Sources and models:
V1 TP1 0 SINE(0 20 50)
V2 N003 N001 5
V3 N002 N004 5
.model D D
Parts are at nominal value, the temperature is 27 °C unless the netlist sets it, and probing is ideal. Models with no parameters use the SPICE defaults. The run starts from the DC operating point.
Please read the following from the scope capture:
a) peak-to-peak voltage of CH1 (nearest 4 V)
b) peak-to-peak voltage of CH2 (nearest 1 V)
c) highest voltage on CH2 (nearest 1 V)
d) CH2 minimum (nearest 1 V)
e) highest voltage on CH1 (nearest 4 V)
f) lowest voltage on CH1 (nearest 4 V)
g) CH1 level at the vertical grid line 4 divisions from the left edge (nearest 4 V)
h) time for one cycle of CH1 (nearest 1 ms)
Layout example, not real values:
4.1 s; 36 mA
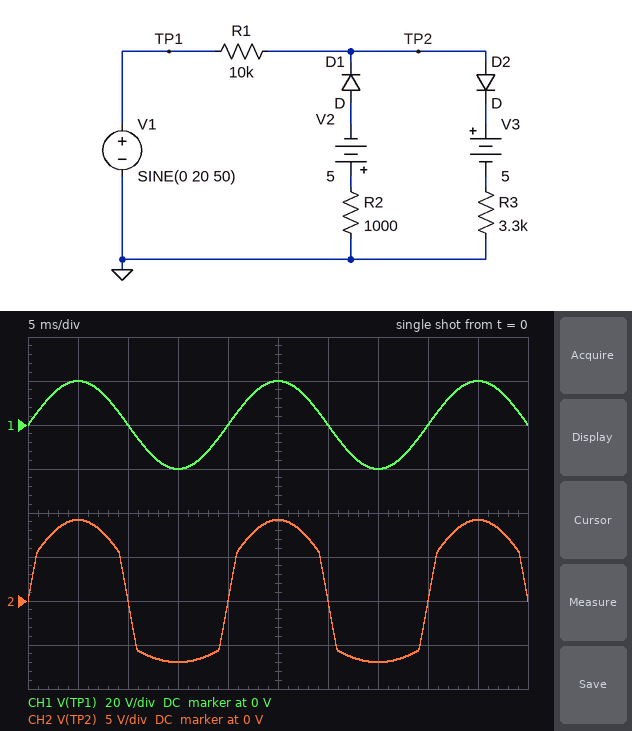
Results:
40 V; 16 V; 9 V; -7 V; 20 V; -20 V; 0 V; 20 ms
